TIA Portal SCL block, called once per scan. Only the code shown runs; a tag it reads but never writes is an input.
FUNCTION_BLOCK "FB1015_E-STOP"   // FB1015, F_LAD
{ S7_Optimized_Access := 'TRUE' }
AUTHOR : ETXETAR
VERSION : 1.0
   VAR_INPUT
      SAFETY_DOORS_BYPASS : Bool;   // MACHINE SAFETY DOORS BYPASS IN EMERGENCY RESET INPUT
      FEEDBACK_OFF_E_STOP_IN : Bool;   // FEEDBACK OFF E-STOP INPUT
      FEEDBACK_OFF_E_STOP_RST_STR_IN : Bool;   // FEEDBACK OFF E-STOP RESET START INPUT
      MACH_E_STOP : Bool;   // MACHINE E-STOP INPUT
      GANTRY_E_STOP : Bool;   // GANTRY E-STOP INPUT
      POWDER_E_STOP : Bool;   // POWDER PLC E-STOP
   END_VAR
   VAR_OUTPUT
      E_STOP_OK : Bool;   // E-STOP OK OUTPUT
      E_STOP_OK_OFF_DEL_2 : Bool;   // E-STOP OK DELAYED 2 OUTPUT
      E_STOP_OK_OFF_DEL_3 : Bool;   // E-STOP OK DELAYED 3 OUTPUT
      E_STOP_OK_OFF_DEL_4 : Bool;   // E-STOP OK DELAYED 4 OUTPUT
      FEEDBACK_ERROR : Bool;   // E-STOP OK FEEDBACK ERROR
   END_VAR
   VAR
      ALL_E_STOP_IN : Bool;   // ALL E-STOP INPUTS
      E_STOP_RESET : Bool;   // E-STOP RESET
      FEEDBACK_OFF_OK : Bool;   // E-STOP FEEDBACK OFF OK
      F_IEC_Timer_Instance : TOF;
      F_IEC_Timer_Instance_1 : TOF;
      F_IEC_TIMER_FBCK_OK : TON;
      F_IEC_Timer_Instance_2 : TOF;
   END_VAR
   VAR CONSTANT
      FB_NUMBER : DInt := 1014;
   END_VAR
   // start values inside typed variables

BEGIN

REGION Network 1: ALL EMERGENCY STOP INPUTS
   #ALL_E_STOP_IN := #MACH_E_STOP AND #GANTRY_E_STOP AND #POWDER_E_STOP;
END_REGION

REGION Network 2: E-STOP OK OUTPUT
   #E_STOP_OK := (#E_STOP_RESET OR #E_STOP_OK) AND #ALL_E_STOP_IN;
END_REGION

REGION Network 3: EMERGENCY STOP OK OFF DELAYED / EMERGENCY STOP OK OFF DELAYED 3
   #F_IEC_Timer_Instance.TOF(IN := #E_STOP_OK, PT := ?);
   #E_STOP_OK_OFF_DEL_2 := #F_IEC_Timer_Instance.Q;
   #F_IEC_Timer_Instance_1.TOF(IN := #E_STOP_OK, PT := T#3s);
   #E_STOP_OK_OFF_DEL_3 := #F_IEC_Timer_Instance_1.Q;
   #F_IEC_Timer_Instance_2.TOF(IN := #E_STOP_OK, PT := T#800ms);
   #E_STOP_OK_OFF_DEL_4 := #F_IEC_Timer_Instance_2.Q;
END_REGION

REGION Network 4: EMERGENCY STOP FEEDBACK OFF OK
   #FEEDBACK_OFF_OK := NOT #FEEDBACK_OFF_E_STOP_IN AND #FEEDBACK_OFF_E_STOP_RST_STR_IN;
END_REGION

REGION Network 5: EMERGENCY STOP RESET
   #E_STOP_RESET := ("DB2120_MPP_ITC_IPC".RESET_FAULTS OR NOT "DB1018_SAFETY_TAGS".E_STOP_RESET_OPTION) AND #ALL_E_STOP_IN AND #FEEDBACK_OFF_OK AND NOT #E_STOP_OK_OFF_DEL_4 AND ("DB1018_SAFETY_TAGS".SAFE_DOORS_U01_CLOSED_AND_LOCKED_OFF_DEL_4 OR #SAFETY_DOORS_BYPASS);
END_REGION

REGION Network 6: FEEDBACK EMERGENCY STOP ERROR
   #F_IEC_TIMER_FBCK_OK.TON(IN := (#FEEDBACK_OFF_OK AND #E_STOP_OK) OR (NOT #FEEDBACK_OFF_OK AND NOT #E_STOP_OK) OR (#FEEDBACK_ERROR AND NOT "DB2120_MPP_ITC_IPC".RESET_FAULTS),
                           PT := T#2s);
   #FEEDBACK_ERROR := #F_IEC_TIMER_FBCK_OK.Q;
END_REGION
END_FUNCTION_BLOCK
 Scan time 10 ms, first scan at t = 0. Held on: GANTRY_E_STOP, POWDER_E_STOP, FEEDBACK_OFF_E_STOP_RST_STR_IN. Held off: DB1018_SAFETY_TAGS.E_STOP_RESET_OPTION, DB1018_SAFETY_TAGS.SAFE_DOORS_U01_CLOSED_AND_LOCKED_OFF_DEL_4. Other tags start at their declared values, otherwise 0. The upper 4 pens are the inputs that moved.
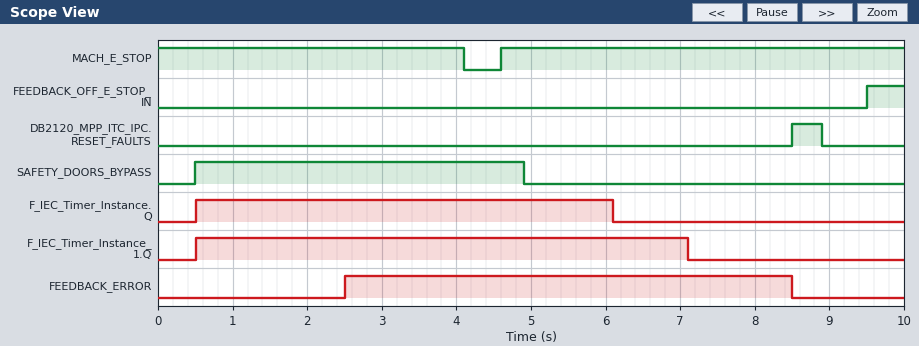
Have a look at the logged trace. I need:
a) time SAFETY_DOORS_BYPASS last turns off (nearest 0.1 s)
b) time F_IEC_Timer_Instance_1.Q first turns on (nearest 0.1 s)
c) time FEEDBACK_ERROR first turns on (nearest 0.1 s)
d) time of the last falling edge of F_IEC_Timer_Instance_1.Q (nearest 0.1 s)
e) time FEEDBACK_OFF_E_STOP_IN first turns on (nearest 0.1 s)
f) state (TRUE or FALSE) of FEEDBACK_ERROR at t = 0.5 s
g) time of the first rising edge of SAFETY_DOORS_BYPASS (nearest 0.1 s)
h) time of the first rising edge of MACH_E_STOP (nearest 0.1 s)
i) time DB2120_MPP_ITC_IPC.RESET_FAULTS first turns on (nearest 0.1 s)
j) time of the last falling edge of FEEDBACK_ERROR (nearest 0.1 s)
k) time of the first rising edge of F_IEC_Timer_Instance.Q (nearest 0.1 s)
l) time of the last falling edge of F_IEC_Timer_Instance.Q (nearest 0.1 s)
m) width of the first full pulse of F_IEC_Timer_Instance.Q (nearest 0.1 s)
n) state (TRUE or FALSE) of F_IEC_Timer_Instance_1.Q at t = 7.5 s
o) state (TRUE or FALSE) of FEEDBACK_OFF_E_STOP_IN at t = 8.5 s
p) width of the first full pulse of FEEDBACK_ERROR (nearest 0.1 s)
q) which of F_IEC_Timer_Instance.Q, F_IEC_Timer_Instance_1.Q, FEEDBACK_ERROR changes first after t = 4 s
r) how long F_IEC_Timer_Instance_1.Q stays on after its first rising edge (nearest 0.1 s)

4.9 s
0.5 s
2.5 s
7.1 s
9.5 s
FALSE
0.5 s
4.6 s
8.5 s
8.5 s
0.5 s
6.1 s
5.6 s
FALSE
FALSE
6.0 s
F_IEC_Timer_Instance.Q
6.6 s
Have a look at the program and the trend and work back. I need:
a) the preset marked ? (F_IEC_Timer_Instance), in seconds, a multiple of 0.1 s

2.0 s
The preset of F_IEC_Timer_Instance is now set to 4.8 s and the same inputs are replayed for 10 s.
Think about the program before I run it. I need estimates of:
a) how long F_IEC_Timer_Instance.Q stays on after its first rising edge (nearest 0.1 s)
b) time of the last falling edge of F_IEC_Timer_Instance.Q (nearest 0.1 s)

8.4 s
8.9 s
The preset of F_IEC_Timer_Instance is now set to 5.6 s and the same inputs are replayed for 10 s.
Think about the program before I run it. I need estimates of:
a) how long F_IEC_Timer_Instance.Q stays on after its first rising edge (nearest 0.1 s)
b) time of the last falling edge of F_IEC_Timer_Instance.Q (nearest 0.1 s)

9.2 s
9.7 s
